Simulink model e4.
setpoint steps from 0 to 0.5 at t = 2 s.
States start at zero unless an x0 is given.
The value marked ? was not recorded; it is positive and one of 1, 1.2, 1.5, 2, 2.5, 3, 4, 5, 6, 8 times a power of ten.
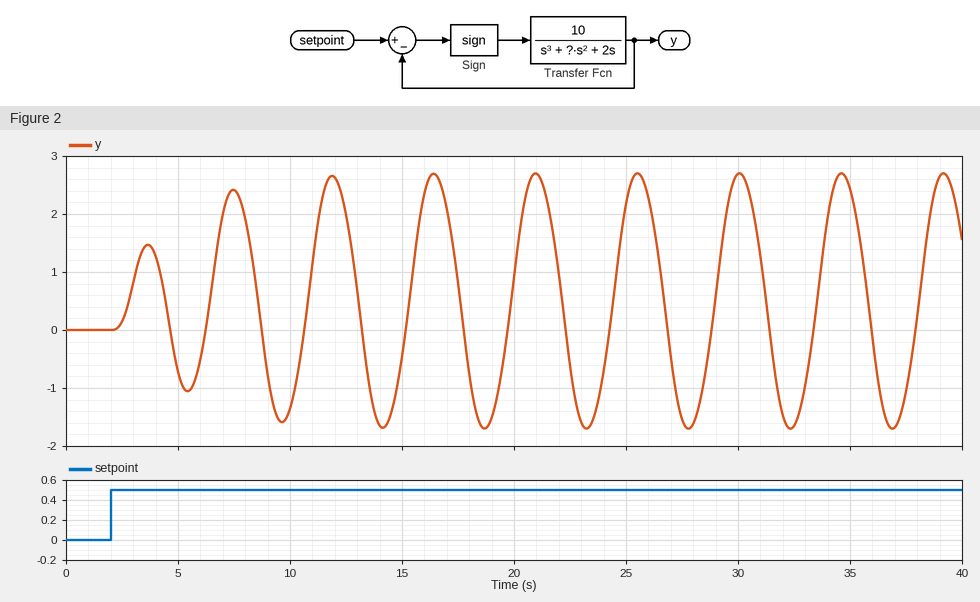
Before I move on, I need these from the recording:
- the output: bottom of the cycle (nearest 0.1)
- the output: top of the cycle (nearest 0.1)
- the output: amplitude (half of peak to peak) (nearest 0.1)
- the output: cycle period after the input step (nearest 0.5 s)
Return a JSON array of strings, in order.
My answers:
["-1.7", "2.7", "2.2", "4.5 s"]
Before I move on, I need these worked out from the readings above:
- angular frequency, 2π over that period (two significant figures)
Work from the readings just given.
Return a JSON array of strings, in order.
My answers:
["1.4 rad/s"]
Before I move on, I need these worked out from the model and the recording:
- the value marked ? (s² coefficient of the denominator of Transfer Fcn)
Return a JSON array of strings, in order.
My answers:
["3"]
